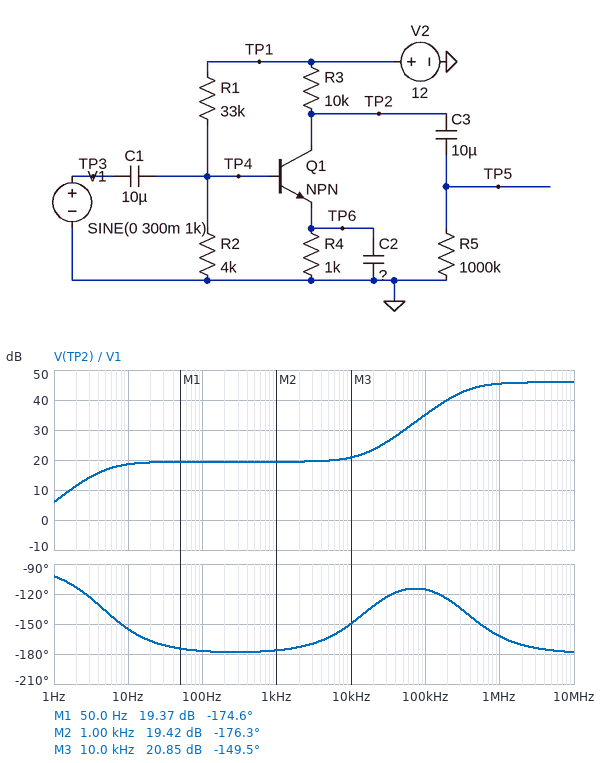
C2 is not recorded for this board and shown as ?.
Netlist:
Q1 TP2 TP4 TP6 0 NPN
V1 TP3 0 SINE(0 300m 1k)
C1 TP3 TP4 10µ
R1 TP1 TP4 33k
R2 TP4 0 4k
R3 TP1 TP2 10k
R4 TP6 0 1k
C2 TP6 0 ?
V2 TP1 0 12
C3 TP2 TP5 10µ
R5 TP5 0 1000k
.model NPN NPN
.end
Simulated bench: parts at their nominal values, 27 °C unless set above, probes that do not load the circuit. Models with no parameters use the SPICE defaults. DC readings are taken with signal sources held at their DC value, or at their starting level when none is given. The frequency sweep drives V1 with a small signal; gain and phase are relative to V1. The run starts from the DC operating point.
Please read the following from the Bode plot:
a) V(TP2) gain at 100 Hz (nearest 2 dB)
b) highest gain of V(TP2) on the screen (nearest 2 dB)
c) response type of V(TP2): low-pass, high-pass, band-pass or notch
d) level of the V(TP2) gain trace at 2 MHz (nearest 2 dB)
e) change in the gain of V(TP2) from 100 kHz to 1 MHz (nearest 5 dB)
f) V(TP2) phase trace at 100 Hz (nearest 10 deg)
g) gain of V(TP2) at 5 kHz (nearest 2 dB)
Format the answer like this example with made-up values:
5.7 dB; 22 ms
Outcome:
20 dB; 46 dB; high-pass; 46 dB; 10 dB; -180 deg; 20 dB
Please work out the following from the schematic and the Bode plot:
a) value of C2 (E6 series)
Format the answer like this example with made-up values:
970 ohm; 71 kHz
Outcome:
10 nF
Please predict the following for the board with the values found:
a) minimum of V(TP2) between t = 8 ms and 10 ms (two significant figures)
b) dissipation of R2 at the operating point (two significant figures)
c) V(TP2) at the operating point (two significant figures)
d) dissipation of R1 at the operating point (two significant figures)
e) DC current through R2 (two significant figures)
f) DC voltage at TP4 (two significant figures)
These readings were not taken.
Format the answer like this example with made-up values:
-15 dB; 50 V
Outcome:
4.0 V; 410 µW; 6.8 V; 3.5 mW; 320 µA; 1.3 V
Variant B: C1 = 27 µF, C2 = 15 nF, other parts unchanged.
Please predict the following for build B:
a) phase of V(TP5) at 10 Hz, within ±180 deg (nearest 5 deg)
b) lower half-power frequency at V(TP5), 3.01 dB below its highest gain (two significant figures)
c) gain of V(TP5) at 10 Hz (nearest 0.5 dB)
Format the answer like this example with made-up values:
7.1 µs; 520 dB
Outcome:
-170 deg; 220 kHz; 19.5 dB
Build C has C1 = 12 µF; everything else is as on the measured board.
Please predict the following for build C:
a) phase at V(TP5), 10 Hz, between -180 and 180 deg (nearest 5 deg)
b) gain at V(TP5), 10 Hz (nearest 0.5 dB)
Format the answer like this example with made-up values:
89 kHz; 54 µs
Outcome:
-160 deg; 19.0 dB
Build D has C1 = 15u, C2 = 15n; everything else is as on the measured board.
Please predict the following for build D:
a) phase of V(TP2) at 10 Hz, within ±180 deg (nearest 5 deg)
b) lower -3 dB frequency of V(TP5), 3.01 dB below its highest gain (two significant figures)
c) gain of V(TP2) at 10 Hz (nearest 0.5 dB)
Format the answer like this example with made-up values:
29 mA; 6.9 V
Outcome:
-165 deg; 220 kHz; 19.0 dB
